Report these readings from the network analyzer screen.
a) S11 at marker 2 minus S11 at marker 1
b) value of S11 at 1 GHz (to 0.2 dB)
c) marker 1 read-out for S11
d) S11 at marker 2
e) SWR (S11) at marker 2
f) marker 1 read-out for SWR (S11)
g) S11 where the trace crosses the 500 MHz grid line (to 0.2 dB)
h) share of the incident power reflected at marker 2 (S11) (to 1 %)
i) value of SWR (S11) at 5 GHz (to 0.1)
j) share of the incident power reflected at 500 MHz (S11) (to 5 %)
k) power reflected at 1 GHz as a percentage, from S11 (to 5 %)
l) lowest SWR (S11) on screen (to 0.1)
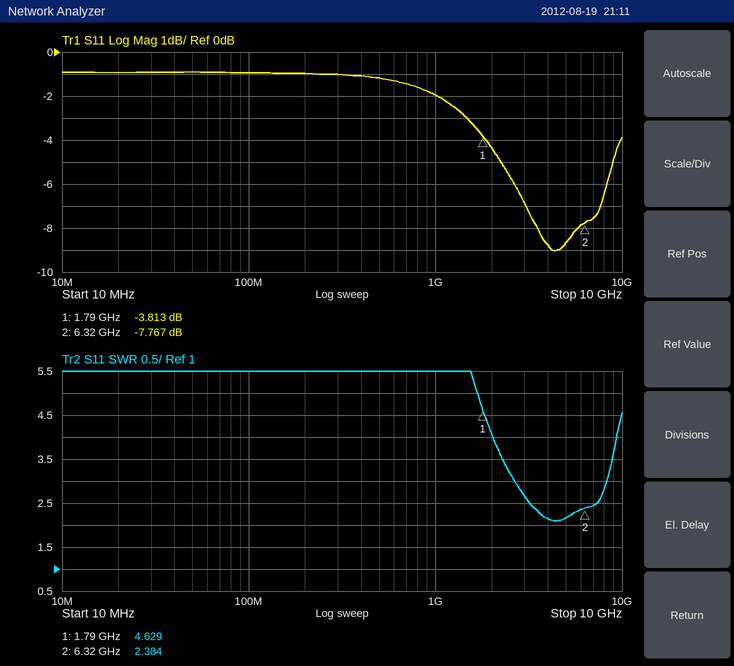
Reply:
-3.954 dB
-2.0 dB
-3.813 dB
-7.767 dB
2.384
4.629
-1.2 dB
17 %
2.2
75 %
65 %
2.1
